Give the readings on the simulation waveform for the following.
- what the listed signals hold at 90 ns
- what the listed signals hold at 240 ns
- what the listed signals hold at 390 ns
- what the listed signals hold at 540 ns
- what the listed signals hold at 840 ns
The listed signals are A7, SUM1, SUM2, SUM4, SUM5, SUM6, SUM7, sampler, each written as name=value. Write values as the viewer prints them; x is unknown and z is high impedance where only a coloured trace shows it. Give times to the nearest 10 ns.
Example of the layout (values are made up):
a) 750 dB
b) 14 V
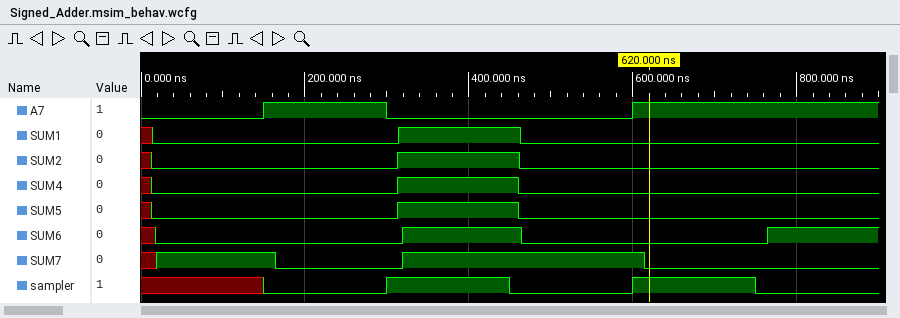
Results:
a) A7=0, SUM1=0, SUM2=0, SUM4=0, SUM5=0, SUM6=0, SUM7=1, sampler=x
b) A7=1, SUM1=0, SUM2=0, SUM4=0, SUM5=0, SUM6=0, SUM7=0, sampler=0
c) A7=0, SUM1=1, SUM2=1, SUM4=1, SUM5=1, SUM6=1, SUM7=1, sampler=1
d) A7=0, SUM1=0, SUM2=0, SUM4=0, SUM5=0, SUM6=0, SUM7=1, sampler=0
e) A7=1, SUM1=0, SUM2=0, SUM4=0, SUM5=0, SUM6=1, SUM7=0, sampler=0
